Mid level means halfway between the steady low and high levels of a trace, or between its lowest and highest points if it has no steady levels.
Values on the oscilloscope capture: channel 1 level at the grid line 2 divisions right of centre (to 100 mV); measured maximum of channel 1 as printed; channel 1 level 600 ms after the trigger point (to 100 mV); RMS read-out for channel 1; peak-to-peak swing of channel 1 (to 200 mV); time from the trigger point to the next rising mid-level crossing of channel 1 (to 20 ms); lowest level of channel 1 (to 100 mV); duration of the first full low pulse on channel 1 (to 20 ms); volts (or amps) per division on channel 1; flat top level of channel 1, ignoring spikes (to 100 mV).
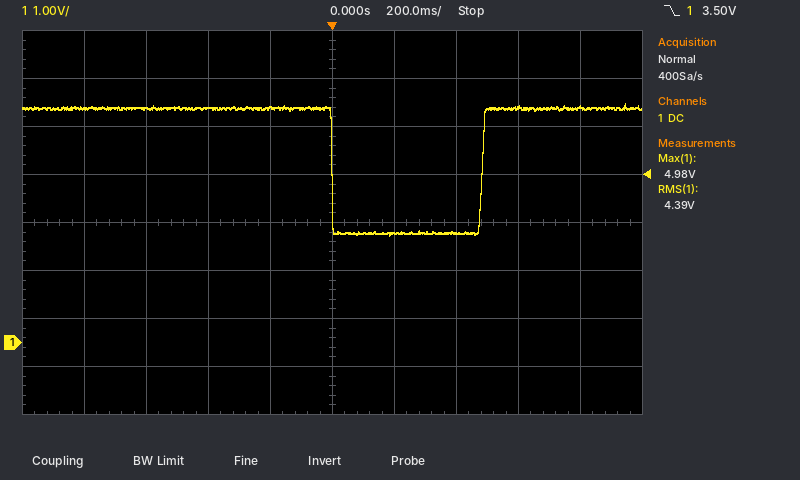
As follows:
2.3 V
4.98 V
4.9 V
4.39 V
2.8 V
480 ms
2.2 V
480 ms
1 V
4.9 V
